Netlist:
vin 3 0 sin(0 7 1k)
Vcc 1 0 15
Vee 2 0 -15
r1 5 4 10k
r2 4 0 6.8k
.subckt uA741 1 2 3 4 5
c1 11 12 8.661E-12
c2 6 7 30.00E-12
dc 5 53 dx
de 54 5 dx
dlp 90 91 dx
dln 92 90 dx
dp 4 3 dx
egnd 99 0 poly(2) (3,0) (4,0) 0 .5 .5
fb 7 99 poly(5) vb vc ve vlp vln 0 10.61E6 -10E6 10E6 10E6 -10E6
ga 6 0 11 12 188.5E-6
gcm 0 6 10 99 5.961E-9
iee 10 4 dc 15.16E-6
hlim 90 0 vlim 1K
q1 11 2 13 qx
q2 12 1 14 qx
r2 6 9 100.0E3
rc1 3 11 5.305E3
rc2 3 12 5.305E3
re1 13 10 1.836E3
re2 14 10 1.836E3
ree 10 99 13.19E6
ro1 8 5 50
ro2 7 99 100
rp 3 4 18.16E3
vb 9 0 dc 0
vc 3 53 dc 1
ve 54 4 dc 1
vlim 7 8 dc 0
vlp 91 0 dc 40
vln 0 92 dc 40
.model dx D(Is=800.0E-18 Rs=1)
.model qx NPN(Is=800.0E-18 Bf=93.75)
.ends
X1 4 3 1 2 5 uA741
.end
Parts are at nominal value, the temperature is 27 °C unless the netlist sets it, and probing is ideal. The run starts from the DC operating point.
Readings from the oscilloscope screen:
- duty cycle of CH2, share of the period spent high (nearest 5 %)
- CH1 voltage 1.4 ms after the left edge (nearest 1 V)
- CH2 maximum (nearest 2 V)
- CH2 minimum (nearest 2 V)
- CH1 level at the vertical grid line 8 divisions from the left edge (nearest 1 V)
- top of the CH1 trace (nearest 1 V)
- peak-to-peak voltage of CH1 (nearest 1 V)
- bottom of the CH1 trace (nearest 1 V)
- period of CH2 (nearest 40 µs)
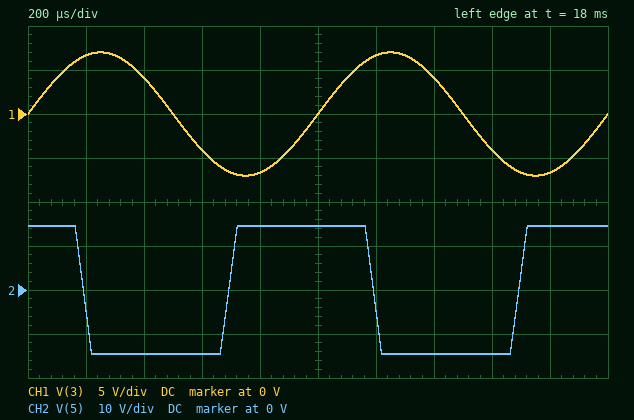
50 %
4 V
14 V
-14 V
-4 V
7 V
14 V
-7 V
1.00 ms
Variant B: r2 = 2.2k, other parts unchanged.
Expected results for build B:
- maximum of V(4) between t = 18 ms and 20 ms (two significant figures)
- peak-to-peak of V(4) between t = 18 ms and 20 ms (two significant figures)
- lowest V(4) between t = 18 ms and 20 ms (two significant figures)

2.6 V
5.3 V
-2.6 V
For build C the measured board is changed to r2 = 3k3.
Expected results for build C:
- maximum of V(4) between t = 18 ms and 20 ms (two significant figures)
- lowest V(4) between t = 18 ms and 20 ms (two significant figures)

3.6 V
-3.6 V
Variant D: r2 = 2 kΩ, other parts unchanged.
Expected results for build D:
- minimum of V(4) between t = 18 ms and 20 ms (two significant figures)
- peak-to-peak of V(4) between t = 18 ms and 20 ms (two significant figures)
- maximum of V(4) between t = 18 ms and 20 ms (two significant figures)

-2.4 V
4.9 V
2.4 V
